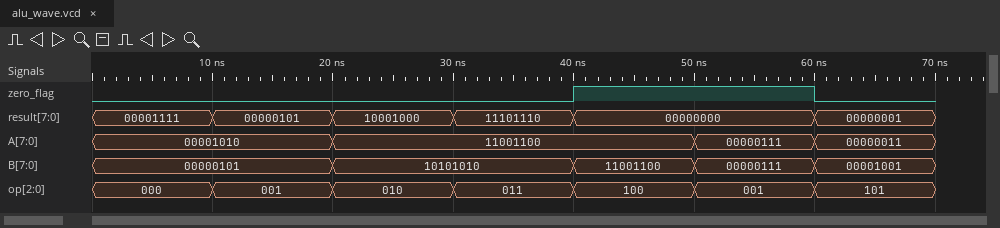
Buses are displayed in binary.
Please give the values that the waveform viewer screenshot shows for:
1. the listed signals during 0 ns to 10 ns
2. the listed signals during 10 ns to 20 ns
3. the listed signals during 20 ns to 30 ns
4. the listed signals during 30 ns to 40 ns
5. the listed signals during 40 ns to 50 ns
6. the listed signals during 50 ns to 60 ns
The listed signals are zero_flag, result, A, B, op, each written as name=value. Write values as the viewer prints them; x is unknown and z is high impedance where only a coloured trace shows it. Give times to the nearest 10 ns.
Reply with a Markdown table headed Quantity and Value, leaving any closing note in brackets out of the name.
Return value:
| Quantity | Value |
|---|---|
| the listed signals during 0 ns to 10 ns | zero_flag=0, result=00001111, A=00001010, B=00000101, op=000 |
| the listed signals during 10 ns to 20 ns | zero_flag=0, result=00000101, A=00001010, B=00000101, op=001 |
| the listed signals during 20 ns to 30 ns | zero_flag=0, result=10001000, A=11001100, B=10101010, op=010 |
| the listed signals during 30 ns to 40 ns | zero_flag=0, result=11101110, A=11001100, B=10101010, op=011 |
| the listed signals during 40 ns to 50 ns | zero_flag=1, result=00000000, A=11001100, B=11001100, op=100 |
| the listed signals during 50 ns to 60 ns | zero_flag=1, result=00000000, A=00000111, B=00000111, op=001 |
